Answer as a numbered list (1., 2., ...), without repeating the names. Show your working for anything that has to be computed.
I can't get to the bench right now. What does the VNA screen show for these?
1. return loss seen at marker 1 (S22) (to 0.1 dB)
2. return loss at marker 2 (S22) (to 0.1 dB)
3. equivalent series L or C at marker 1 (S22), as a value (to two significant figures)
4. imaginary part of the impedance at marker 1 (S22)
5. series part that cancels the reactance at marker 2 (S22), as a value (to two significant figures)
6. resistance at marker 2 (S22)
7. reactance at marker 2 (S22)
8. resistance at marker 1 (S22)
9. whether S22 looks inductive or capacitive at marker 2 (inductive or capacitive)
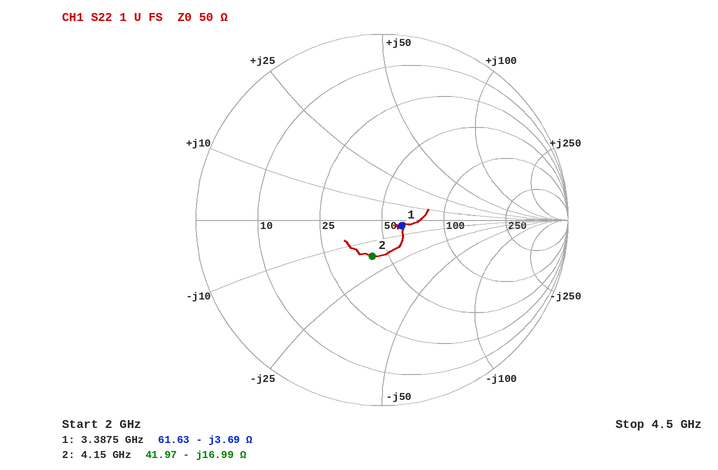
1. 19.2 dB
2. 13.9 dB
3. C = 1/(2π × 3.3875 GHz × 3.69 Ω) ≈ 13 pF
4. -3.69 Ω
5. L = 16.99 Ω/(2π × 4.15 GHz) ≈ 652 pH, so 650 pH to two significant figures
6. 41.97 Ω
7. -16.99 Ω
8. 61.63 Ω
9. capacitive
